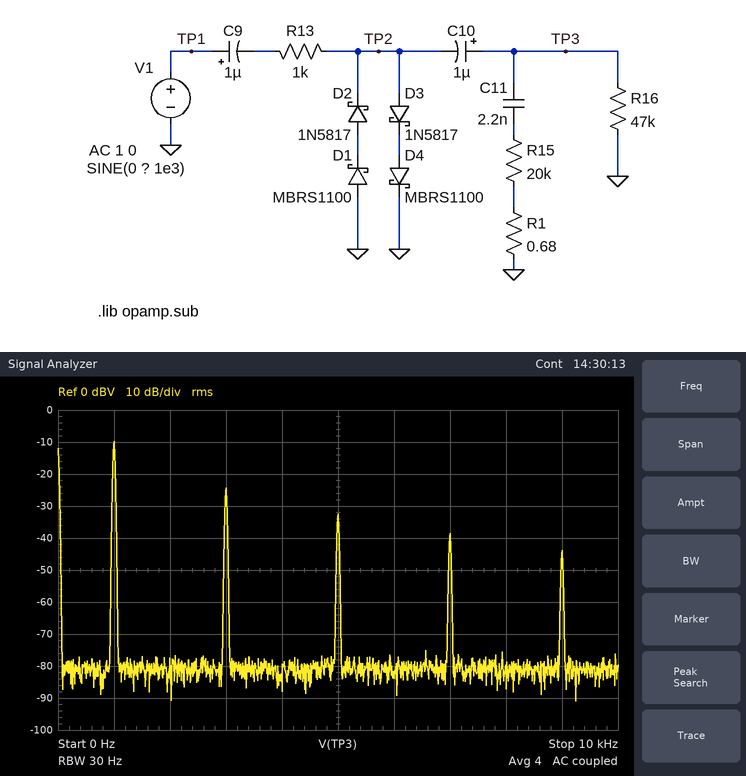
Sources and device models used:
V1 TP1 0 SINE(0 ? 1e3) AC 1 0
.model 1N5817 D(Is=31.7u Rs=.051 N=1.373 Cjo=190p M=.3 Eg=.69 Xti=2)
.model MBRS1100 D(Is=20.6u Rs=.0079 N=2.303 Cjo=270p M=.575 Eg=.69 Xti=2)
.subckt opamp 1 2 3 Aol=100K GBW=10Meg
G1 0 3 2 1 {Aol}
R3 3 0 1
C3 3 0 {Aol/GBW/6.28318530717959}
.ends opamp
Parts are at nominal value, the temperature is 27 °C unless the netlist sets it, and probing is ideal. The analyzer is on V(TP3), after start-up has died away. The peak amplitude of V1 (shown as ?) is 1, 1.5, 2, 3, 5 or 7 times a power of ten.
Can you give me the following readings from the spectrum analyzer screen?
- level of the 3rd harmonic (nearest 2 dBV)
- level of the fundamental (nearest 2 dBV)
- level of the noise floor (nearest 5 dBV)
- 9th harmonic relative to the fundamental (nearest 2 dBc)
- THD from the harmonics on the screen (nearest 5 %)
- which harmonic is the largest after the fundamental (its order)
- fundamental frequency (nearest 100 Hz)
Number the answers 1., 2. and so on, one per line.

1. -24 dBV
2. -10 dBV
3. -80 dBV
4. -34 dBc
5. 20 %
6. 3
7. 1.0 kHz
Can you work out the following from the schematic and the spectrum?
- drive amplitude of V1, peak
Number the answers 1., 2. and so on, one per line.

1. 2 V
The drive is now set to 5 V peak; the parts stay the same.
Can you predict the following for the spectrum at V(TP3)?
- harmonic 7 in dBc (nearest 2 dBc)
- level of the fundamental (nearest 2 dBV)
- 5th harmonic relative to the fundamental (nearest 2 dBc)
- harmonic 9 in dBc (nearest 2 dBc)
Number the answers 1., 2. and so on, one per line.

1. -24 dBc
2. -8 dBV
3. -20 dBc
4. -28 dBc
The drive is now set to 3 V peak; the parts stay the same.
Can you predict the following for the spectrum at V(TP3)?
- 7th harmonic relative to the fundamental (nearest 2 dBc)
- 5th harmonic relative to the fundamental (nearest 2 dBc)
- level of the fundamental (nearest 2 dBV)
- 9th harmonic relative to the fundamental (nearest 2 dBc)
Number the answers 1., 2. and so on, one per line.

1. -26 dBc
2. -20 dBc
3. -8 dBV
4. -30 dBc
